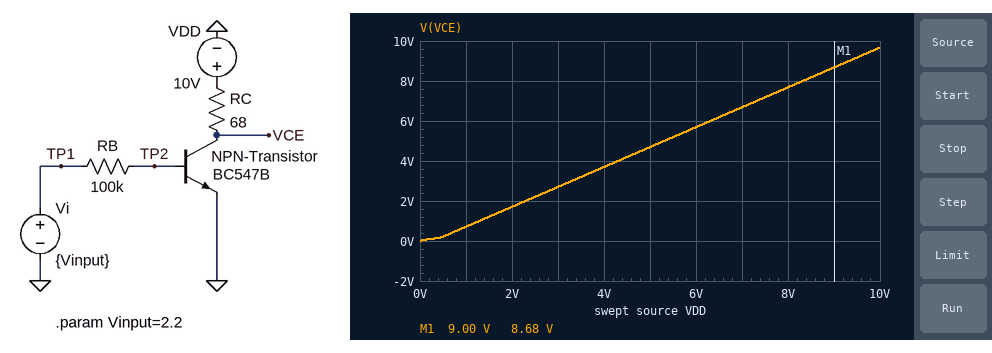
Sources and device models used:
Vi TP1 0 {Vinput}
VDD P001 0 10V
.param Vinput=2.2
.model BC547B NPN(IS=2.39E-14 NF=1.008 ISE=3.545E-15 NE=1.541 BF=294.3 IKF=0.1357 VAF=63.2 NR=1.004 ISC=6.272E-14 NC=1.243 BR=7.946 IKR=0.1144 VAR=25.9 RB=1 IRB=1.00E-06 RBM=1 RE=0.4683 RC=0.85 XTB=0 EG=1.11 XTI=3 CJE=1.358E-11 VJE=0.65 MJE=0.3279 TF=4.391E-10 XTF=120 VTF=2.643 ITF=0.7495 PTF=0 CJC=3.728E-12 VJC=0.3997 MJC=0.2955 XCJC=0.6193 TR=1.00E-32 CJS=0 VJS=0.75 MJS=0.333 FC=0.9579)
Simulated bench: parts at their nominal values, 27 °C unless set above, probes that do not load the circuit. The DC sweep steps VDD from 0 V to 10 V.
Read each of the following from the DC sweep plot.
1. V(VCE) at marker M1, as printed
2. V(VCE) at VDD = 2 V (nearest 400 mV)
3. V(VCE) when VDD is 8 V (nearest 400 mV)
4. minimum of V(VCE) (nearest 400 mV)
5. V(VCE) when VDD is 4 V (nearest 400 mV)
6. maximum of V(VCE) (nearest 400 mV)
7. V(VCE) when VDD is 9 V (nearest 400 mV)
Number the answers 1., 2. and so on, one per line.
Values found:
1. 8.68 V
2. 1.6 V
3. 7.6 V
4. 0 V
5. 3.6 V
6. 9.6 V
7. 8.8 V
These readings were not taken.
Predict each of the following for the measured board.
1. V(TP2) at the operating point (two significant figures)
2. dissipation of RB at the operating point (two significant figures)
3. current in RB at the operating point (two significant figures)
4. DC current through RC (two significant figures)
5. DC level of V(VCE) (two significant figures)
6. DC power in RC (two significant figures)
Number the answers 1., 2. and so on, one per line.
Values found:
1. 680 mV
2. 23 µW
3. 15 µA
4. 4.8 mA
5. 9.7 V
6. 1.6 mW
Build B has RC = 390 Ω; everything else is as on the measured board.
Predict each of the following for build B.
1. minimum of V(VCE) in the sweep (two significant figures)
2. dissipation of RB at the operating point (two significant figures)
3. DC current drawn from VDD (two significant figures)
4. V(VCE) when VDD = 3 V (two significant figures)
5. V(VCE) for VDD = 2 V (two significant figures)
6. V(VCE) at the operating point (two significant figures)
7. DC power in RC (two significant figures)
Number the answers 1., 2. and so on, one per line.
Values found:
1. 3.9 mV
2. 23 µW
3. 4.7 mA
4. 1.3 V
5. 370 mV
6. 8.2 V
7. 8.7 mW
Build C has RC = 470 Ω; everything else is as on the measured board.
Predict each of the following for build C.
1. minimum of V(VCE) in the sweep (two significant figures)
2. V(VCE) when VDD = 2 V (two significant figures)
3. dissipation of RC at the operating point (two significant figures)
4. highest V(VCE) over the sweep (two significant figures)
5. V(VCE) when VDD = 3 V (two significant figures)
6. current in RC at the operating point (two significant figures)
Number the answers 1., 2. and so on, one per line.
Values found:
1. 4.2 mV
2. 180 mV
3. 10 mW
4. 7.8 V
5. 1.0 V
6. 4.7 mA
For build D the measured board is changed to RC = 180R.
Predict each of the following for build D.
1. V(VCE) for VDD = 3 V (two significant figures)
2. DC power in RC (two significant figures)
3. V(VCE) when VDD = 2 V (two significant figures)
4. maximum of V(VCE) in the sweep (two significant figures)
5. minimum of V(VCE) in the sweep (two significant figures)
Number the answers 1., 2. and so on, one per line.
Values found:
1. 2.2 V
2. 4.1 mW
3. 1.2 V
4. 9.1 V
5. 2.6 mV
